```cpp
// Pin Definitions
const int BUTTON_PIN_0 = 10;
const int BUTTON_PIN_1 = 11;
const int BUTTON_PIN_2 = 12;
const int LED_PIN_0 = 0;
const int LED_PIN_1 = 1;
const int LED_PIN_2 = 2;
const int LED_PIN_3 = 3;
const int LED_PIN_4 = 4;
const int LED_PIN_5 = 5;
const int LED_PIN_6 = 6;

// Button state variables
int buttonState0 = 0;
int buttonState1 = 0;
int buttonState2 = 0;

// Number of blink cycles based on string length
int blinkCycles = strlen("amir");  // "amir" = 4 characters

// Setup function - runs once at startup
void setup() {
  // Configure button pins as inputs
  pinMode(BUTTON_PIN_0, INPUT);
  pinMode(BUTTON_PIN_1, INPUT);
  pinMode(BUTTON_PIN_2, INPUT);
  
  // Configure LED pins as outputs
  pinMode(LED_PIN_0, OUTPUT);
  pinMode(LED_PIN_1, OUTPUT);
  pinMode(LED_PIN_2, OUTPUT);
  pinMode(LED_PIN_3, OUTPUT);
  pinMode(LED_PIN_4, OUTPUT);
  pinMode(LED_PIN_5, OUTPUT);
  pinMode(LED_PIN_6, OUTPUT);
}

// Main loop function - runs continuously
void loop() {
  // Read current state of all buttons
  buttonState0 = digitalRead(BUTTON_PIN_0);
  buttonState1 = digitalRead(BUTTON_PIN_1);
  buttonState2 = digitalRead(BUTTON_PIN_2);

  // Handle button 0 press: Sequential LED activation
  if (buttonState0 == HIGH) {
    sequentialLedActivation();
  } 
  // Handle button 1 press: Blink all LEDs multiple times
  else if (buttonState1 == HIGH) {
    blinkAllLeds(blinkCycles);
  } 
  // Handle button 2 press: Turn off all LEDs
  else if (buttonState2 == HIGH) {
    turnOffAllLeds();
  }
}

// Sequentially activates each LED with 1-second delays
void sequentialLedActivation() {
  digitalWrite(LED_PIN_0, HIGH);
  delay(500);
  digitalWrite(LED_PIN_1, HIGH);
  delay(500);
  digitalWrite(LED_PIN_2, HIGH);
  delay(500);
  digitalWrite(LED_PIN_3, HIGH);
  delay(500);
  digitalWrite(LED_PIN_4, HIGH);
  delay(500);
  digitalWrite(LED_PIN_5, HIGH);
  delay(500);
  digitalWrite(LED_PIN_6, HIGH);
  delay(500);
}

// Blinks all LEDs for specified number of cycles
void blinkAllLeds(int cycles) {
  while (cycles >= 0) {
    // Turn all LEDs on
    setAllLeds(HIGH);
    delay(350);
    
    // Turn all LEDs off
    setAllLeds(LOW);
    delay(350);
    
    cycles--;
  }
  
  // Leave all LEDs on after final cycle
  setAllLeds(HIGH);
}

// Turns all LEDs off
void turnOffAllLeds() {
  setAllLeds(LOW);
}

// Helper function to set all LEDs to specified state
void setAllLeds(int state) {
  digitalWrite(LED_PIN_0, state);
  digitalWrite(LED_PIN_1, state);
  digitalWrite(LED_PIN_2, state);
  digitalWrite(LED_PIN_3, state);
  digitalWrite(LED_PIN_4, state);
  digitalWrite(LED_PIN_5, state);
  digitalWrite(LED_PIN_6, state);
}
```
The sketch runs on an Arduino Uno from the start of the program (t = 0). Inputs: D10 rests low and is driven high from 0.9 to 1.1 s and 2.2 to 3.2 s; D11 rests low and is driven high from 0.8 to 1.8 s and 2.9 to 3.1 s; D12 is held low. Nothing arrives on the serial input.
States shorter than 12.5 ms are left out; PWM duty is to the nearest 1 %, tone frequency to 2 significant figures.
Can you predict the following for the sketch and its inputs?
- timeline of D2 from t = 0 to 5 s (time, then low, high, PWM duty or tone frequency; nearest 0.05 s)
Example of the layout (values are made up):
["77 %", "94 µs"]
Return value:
["0 s low; 0.8 s high; 1.15 s low; 1.5 s high; 1.85 s low; 2.2 s high; 2.55 s low; 2.9 s high; 3.25 s low; 3.6 s high; 3.95 s low; 4.3 s high"]
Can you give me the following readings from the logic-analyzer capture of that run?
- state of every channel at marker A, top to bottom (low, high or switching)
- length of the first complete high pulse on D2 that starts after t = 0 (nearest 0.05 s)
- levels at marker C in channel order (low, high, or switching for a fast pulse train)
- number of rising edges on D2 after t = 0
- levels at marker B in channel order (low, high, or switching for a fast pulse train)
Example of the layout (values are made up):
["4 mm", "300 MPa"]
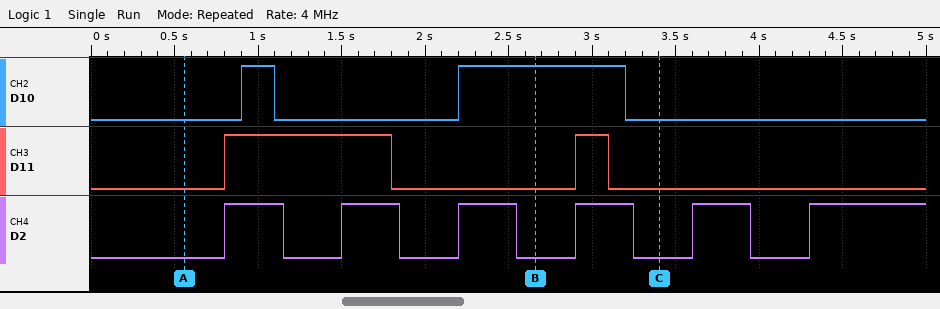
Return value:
["D10 low, D11 low, D2 low", "0.35 s", "D10 low, D11 low, D2 low", "6", "D10 high, D11 low, D2 low"]
